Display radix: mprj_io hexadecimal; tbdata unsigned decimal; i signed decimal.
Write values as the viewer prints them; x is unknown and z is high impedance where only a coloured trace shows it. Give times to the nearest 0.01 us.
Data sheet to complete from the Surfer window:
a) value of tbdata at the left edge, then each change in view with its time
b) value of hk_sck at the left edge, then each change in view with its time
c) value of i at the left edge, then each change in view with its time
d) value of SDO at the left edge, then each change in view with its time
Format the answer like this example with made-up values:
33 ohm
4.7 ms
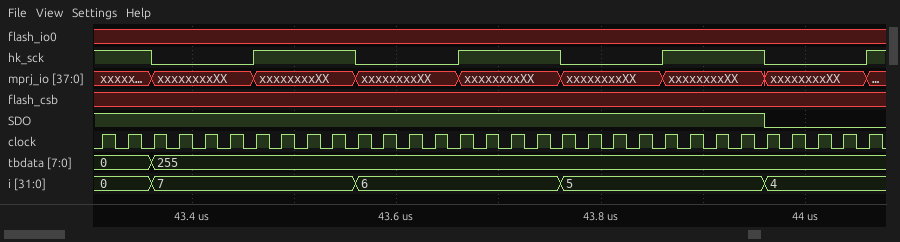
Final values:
0, 255 at 43.36 us
1, 0 at 43.36 us, 1 at 43.46 us, 0 at 43.56 us, 1 at 43.66 us, 0 at 43.76 us, 1 at 43.86 us, 0 at 43.96 us, 1 at 44.06 us
0, 7 at 43.36 us, 6 at 43.56 us, 5 at 43.76 us, 4 at 43.96 us
1, 0 at 43.96 us
